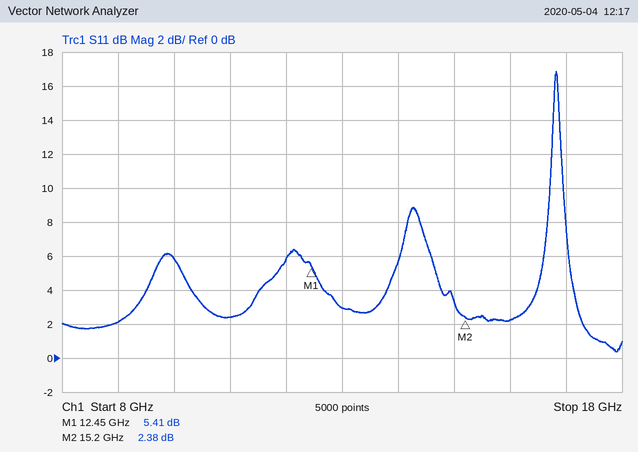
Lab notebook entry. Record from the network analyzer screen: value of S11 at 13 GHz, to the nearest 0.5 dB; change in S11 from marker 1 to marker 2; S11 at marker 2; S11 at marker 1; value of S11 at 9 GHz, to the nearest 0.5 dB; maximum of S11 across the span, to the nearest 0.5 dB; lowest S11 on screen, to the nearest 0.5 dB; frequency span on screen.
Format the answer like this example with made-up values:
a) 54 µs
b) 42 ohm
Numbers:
a) 3.0 dB
b) -3.03 dB
c) 2.38 dB
d) 5.41 dB
e) 2.0 dB
f) 17.0 dB
g) 0.5 dB
h) 10 GHz
